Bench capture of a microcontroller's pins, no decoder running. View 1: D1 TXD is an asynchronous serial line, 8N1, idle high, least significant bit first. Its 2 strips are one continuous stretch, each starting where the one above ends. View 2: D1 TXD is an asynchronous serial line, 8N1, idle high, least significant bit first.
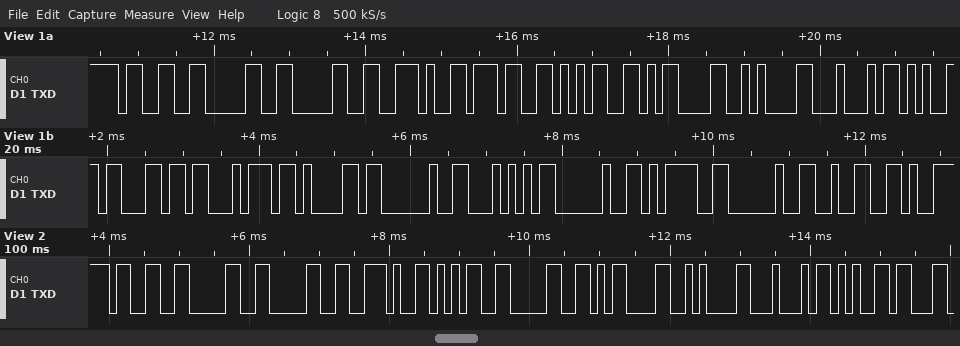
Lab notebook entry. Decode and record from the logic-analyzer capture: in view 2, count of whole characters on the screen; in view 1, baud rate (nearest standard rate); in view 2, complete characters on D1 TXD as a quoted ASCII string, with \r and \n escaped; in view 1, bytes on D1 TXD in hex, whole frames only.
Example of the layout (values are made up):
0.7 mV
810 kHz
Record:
10
9600 baud
"300.50\r\nDe"
0x33 0x30 0x30 0x2E 0x37 0x35 0x0D 0x0A 0x44 0x65 0x6C 0x74 0x61 0x20 0x54 0x20 0x3D 0x20 0x32
